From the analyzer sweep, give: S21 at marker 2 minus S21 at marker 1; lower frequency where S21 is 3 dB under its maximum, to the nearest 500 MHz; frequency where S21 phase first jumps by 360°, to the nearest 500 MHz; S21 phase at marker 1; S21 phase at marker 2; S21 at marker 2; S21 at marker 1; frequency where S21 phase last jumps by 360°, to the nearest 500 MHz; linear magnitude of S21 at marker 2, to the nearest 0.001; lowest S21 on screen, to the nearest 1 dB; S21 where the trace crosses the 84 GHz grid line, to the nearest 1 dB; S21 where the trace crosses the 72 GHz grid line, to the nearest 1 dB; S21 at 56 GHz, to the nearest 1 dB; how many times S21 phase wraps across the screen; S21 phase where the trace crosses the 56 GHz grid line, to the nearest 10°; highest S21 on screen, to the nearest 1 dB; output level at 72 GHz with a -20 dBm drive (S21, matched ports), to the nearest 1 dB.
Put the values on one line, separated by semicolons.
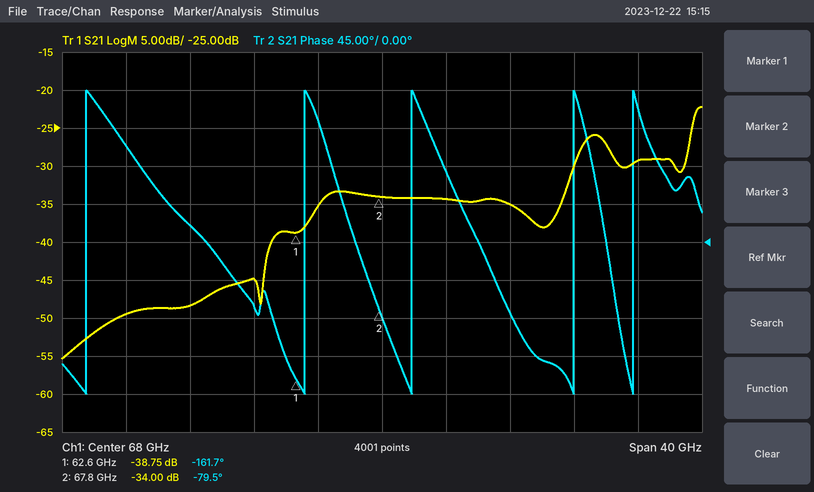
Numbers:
4.75 dB; 87.5 GHz; 49.5 GHz; -161.7°; -79.5°; -34.00 dB; -38.75 dB; 83.5 GHz; 0.020; -55 dB; -29 dB; -34 dB; -48 dB; 5; 20°; -22 dB; -54 dBm
